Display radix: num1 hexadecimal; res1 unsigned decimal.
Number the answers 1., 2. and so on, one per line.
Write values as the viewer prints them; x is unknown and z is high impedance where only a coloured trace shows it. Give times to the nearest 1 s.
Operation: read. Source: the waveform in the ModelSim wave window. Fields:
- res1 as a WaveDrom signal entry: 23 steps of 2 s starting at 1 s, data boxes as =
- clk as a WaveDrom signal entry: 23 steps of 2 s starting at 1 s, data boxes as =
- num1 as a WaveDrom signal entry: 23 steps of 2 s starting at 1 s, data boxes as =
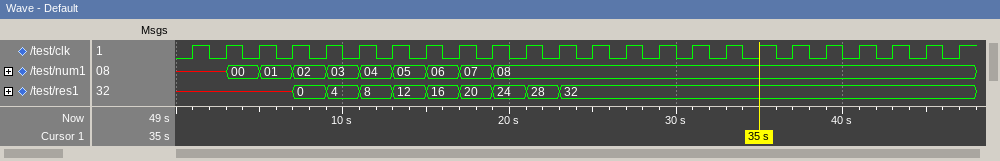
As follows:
1. {name: 'res1', wave: 'x..=========...........', data: '0 4 8 12 16 20 24 28 32'}
2. {name: 'clk', wave: 'p......................'}
3. {name: 'num1', wave: 'x=========.............', data: '00 01 02 03 04 05 06 07 08'}
